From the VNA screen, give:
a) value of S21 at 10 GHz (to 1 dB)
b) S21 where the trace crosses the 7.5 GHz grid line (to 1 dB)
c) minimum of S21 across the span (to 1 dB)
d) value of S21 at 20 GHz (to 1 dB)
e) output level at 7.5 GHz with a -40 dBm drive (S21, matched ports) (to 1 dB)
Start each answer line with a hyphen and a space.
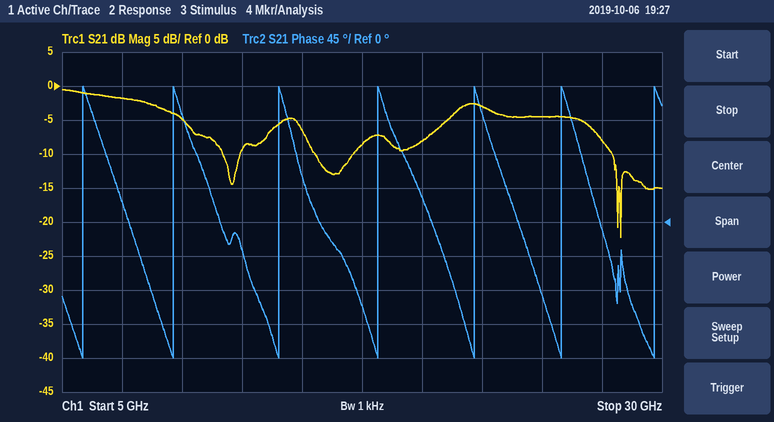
- -5 dB
- -2 dB
- -22 dB
- -8 dB
- -42 dBm
